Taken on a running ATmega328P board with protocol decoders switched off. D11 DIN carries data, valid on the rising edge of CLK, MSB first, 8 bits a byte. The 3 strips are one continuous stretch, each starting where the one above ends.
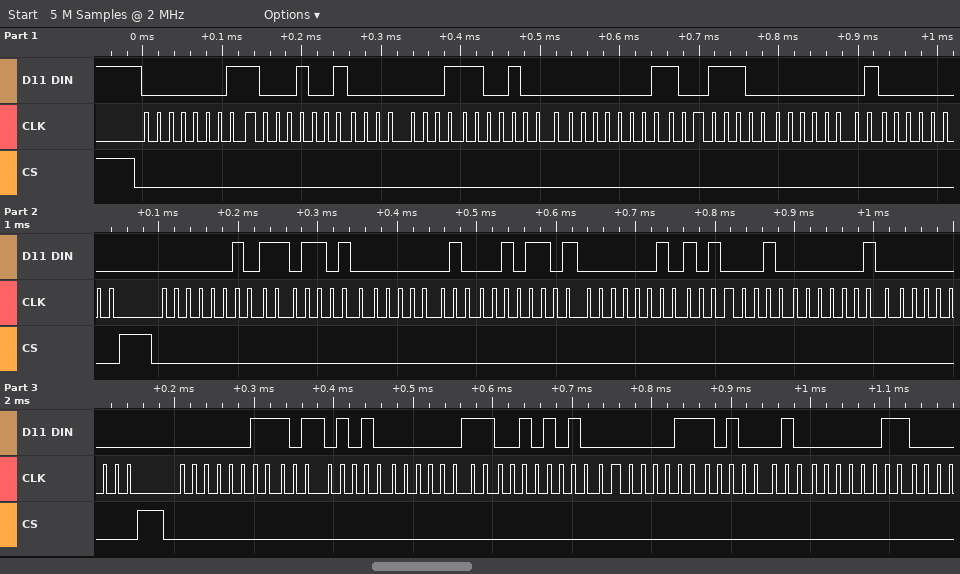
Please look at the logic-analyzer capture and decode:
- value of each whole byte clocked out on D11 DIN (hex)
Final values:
01 89 01 C8 01 9C 01 00 02 DA 02 2D 02 A2 02 00 03 AA 03 2A 03 A2 03
